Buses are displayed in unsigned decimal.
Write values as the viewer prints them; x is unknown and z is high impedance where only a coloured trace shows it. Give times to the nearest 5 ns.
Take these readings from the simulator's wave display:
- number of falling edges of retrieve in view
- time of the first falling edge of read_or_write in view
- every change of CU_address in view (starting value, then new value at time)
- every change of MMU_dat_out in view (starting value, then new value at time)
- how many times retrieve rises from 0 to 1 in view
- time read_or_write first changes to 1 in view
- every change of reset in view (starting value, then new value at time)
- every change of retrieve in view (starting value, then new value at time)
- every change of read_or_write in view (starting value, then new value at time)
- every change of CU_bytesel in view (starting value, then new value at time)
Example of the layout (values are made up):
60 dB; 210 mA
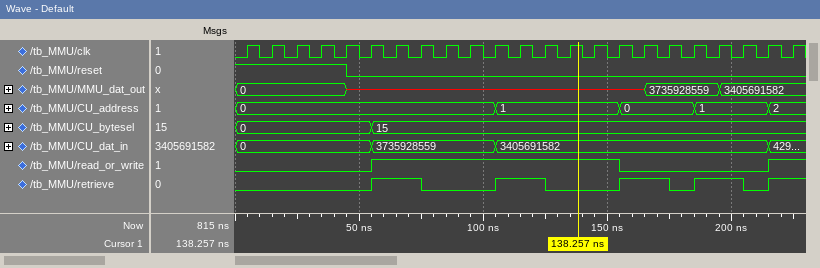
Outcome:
4; 155 ns; 0, 1 at 105 ns, 0 at 155 ns, 1 at 185 ns, 2 at 215 ns; 0, x at 45 ns, 3735928559 at 165 ns, 3405691582 at 195 ns; 5; 55 ns; 1, 0 at 45 ns; 0, 1 at 55 ns, 0 at 75 ns, 1 at 105 ns, 0 at 125 ns, 1 at 155 ns, 0 at 175 ns, 1 at 185 ns, 0 at 205 ns, 1 at 215 ns; 0, 1 at 55 ns, 0 at 155 ns, 1 at 215 ns; 0, 15 at 55 ns
